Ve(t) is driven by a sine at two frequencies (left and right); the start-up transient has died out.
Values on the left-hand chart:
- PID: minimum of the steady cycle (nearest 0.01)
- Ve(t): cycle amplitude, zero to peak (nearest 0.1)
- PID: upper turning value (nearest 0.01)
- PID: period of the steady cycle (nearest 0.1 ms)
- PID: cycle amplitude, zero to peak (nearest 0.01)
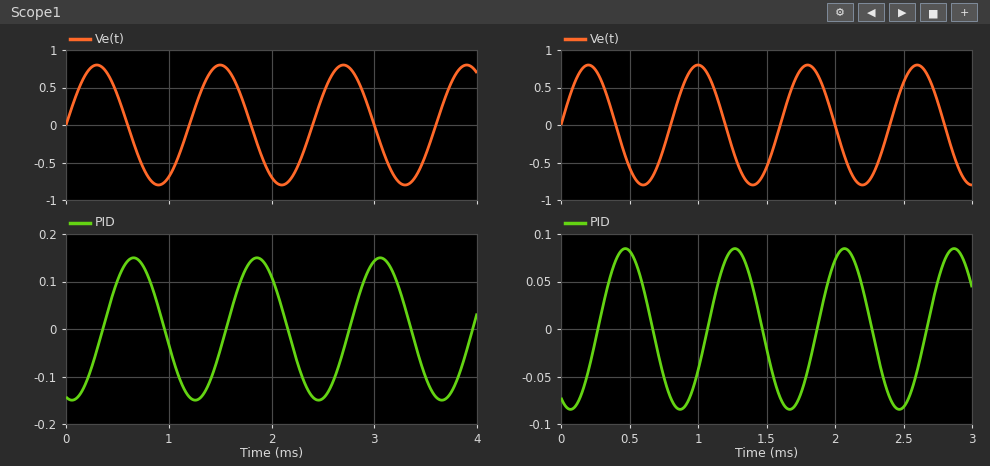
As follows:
-0.15
0.8
0.15
1.2 ms
0.15
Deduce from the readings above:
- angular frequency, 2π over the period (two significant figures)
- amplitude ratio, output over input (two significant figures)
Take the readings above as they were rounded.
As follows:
5.2 rad/ms
0.19
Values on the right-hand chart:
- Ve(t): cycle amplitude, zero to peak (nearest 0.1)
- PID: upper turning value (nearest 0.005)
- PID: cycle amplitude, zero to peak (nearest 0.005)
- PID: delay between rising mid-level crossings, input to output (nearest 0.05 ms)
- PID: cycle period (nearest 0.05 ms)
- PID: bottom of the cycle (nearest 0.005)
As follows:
0.8
0.085
0.085
0.25 ms
0.80 ms
-0.085
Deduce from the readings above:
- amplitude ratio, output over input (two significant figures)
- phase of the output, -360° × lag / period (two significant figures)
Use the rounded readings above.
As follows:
0.11
-110°
